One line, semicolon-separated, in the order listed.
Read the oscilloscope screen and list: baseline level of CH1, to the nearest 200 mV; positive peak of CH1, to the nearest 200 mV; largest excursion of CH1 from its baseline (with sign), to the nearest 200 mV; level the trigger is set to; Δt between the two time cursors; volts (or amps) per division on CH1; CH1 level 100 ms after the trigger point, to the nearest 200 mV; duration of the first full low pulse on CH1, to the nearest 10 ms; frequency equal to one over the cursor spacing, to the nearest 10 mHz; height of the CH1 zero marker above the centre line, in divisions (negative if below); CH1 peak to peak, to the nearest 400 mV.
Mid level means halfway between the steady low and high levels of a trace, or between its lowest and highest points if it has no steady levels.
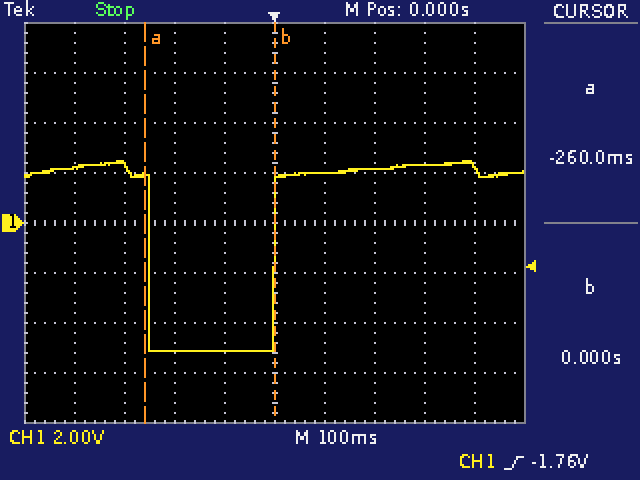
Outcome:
2.0 V; 2.4 V; -7.2 V; -1.76 V; 260 ms; 2 V; 2.0 V; 250 ms; 3.85 Hz; 0.0 div; 7.6 V
